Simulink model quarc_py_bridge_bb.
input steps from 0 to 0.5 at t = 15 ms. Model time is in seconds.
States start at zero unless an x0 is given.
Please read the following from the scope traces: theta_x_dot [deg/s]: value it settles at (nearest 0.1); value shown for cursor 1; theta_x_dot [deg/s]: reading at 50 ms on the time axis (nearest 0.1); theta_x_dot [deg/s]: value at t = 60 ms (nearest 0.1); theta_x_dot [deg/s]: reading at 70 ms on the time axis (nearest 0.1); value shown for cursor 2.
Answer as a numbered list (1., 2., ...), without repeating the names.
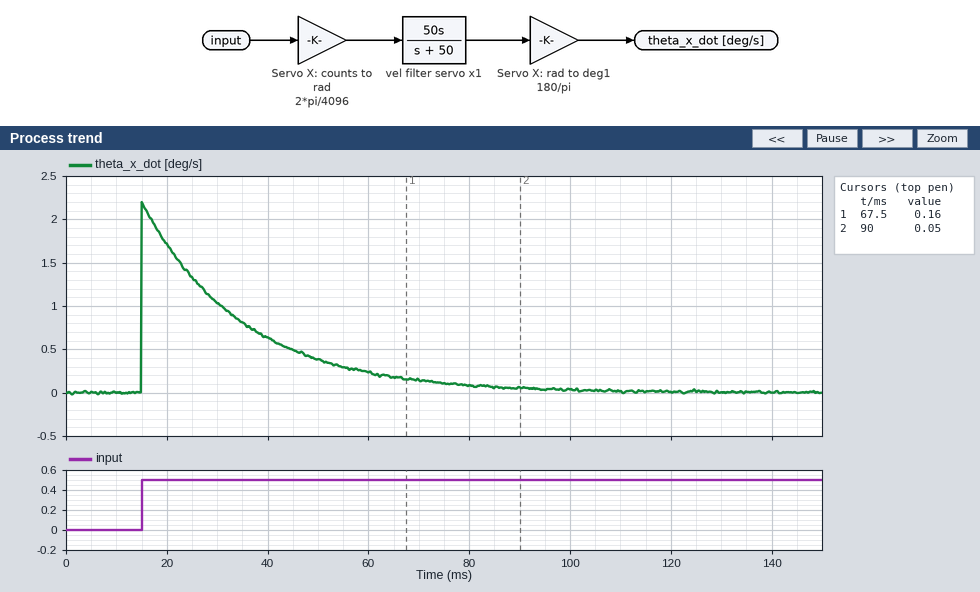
1. 0.0
2. 0.16
3. 0.4
4. 0.2
5. 0.1
6. 0.05
